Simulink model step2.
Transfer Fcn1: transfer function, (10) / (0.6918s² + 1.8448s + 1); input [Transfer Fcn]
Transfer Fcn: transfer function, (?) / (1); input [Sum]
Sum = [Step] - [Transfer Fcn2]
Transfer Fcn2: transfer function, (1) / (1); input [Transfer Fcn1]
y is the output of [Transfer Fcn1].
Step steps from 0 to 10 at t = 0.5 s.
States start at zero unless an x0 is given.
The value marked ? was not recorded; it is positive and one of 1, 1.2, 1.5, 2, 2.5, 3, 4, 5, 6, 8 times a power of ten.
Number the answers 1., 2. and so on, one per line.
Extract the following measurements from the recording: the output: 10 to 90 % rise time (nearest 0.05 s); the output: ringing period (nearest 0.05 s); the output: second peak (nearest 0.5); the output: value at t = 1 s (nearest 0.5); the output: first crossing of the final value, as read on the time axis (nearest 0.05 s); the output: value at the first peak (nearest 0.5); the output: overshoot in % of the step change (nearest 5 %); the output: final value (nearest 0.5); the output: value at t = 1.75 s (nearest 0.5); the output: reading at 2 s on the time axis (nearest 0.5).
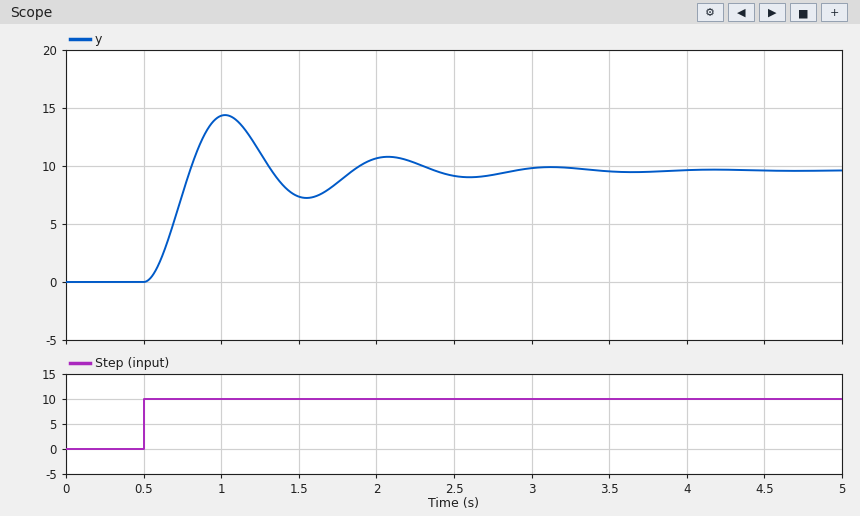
1. 0.20 s
2. 1.05 s
3. 11.0
4. 14.5
5. 0.80 s
6. 14.5
7. 50 %
8. 9.5
9. 8.5
10. 10.5
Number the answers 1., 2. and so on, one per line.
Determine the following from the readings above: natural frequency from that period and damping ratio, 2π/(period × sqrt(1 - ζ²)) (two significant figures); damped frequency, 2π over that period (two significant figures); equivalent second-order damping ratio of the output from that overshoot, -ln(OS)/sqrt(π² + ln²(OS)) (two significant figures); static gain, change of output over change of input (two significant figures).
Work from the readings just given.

1. 6.1 rad/s
2. 6.0 rad/s
3. 0.22
4. 0.95
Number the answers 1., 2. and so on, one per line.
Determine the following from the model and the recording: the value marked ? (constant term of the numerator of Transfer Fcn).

1. 2.5
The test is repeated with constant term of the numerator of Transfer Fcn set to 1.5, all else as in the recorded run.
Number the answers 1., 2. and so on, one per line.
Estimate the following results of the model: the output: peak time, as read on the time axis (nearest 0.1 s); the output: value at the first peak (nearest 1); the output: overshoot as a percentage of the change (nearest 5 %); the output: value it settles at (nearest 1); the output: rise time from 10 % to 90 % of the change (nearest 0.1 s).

1. 1.2 s
2. 13
3. 40 %
4. 9
5. 0.3 s
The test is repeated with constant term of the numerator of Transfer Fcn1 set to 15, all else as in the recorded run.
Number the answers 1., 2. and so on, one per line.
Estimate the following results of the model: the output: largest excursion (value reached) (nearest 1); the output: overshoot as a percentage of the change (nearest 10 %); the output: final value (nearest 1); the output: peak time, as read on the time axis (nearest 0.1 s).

1. 15
2. 60 %
3. 10
4. 0.9 s
